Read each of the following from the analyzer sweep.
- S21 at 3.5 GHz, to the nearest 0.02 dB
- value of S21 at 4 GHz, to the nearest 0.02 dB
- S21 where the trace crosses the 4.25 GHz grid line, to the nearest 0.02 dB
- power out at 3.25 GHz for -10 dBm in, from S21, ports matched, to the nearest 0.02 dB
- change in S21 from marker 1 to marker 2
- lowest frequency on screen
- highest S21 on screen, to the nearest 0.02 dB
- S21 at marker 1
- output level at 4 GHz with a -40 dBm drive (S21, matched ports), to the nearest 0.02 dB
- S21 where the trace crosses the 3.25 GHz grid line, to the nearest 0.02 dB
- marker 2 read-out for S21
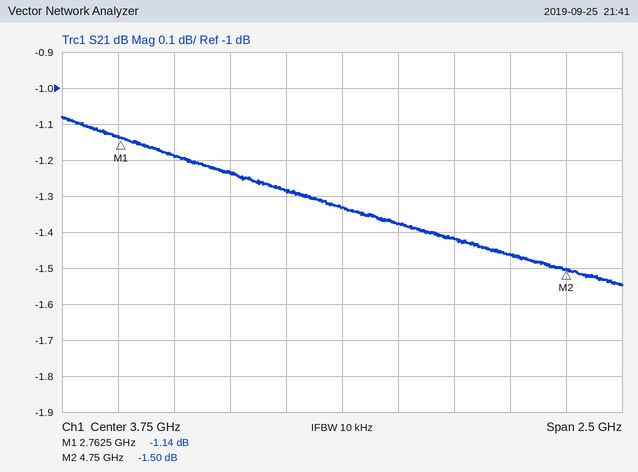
-1.28 dB
-1.38 dB
-1.42 dB
-11.24 dBm
-0.36 dB
2.5 GHz
-1.08 dB
-1.14 dB
-41.38 dBm
-1.24 dB
-1.50 dB
